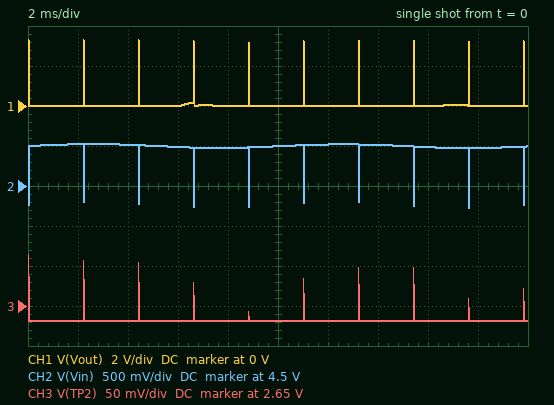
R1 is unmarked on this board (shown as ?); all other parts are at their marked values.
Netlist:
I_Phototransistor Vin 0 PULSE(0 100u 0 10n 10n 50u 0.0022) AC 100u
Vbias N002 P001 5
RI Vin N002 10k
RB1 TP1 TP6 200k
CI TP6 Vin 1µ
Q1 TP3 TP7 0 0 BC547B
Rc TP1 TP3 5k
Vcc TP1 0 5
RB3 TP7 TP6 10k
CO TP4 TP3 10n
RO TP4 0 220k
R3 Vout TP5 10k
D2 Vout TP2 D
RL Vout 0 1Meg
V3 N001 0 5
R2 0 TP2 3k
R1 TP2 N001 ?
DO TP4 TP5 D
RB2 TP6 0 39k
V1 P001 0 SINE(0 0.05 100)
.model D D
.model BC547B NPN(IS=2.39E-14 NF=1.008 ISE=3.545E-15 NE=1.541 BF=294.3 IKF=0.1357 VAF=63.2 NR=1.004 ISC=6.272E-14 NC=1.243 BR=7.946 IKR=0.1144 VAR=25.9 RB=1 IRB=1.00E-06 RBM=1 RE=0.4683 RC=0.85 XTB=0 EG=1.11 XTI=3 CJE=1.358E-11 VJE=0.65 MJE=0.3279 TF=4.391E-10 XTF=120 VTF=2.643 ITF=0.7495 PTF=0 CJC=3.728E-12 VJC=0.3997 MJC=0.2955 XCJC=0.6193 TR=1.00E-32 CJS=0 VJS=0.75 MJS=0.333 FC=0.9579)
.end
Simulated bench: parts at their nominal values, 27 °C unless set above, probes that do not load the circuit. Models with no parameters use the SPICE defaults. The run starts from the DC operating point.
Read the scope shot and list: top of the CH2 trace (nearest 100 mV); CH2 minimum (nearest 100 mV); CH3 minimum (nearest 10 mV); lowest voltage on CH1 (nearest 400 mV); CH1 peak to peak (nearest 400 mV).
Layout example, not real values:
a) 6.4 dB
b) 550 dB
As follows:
a) 5.0 V
b) 4.2 V
c) 2.63 V
d) 0 V
e) 3.2 V
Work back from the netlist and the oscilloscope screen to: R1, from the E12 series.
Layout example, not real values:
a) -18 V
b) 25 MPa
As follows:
a) 2.7 kΩ
